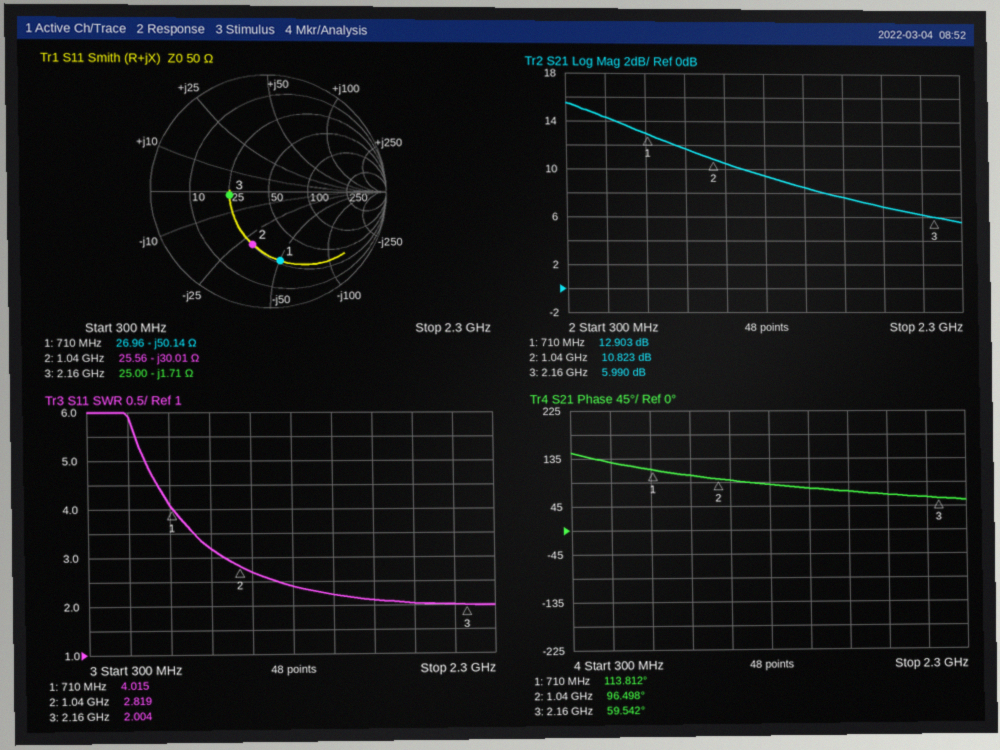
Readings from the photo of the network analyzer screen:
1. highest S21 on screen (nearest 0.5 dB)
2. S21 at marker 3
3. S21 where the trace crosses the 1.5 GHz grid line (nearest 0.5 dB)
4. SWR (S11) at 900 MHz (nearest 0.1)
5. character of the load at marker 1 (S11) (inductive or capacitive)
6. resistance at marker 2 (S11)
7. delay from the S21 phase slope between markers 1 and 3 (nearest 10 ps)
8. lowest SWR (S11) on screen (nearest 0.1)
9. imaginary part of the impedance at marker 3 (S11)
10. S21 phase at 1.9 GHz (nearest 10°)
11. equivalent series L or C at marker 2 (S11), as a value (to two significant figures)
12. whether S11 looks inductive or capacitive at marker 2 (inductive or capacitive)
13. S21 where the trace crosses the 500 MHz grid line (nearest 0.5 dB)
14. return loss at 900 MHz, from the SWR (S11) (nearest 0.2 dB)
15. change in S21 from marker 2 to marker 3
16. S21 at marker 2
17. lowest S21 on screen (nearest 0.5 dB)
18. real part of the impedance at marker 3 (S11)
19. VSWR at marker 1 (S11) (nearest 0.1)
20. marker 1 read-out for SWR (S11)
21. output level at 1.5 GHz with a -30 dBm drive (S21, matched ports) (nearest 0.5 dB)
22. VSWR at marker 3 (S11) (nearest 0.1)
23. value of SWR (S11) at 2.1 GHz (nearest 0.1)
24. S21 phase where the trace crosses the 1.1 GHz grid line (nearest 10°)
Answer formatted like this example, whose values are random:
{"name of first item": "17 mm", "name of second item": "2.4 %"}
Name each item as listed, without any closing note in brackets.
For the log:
{"highest S21 on screen": "15.5 dB", "S21 at marker 3": "5.990 dB", "S21 where the trace crosses the 1.5 GHz grid line": "8.5 dB", "SWR (S11) at 900 MHz": "3.2", "character of the load at marker 1 (S11)": "capacitive", "resistance at marker 2": "25.56 Ω", "delay from the S21 phase slope between markers 1 and 3": "100 ps", "lowest SWR (S11) on screen": "2.0", "imaginary part of the impedance at marker 3": "-1.71 Ω", "S21 phase at 1.9 GHz": "70°", "equivalent series L or C at marker 2 (S11), as a value": "5.1 pF", "whether S11 looks inductive or capacitive at marker 2": "capacitive", "S21 where the trace crosses the 500 MHz grid line": "14.5 dB", "return loss at 900 MHz, from the SWR (S11)": "5.6 dB", "change in S21 from marker 2 to marker 3": "-4.833 dB", "S21 at marker 2": "10.823 dB", "lowest S21 on screen": "5.5 dB", "real part of the impedance at marker 3": "25.00 Ω", "VSWR at marker 1 (S11)": "4.0", "marker 1 read-out for SWR": "4.015", "output level at 1.5 GHz with a -30 dBm drive (S21, matched ports)": "-21.5 dBm", "VSWR at marker 3 (S11)": "2.0", "value of SWR (S11) at 2.1 GHz": "2.0", "S21 phase where the trace crosses the 1.1 GHz grid line": "90°"}
